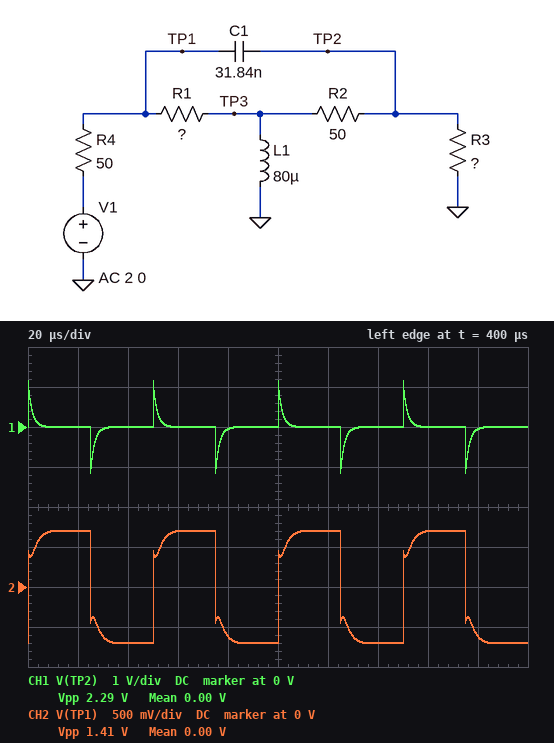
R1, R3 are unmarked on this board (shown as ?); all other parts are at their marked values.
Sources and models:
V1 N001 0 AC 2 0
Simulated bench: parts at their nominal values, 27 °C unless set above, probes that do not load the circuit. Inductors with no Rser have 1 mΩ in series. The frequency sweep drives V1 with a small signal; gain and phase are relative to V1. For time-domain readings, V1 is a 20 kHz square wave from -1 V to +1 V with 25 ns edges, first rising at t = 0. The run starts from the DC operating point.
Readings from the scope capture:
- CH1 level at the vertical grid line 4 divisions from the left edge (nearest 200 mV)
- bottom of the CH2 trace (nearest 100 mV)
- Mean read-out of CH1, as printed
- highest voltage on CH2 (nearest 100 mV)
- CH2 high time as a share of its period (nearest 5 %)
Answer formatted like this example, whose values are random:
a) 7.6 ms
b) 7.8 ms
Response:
a) 0 V
b) -700 mV
c) 0.00 V
d) 700 mV
e) 50 %
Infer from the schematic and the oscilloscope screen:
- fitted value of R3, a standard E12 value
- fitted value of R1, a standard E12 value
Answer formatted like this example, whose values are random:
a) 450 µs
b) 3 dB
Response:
a) 68 Ω
b) 120 Ω
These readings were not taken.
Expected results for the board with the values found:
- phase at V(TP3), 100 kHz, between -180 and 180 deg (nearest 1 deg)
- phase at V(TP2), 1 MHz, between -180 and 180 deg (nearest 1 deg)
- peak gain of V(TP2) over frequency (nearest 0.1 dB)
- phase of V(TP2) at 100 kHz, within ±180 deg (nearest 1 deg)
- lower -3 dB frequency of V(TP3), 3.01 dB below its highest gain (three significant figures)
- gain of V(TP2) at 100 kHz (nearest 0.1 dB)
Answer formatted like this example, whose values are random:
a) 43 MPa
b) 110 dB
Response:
a) 63 deg
b) 6 deg
c) -4.8 dB
d) 45 deg
e) 140 kHz
f) -7.8 dB
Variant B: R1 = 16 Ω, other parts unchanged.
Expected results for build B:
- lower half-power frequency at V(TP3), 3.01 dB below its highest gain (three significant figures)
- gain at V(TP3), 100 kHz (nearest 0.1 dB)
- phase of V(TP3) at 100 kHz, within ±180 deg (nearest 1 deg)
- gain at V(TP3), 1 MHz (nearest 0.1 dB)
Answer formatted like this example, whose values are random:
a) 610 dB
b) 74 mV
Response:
a) 70.9 kHz
b) -6.4 dB
c) 37 deg
d) -4.8 dB
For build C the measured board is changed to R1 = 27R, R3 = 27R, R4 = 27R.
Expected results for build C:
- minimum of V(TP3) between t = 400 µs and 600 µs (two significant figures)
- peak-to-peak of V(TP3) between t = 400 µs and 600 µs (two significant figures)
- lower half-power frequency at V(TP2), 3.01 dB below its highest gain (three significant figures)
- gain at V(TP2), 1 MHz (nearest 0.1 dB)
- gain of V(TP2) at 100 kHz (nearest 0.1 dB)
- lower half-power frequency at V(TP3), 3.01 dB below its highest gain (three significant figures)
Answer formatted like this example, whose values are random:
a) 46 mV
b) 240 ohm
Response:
a) -1.0 V
b) 2.0 V
c) 122 kHz
d) -6.1 dB
e) -9.8 dB
f) 50.2 kHz
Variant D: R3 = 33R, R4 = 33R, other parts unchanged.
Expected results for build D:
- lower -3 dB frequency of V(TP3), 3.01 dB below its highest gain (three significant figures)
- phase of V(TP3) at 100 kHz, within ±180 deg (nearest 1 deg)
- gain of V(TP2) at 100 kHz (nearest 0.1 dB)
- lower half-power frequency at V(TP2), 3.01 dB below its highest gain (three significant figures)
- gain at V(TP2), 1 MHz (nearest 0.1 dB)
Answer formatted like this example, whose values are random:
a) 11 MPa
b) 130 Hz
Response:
a) 131 kHz
b) 57 deg
c) -9.4 dB
d) 108 kHz
e) -6.1 dB
